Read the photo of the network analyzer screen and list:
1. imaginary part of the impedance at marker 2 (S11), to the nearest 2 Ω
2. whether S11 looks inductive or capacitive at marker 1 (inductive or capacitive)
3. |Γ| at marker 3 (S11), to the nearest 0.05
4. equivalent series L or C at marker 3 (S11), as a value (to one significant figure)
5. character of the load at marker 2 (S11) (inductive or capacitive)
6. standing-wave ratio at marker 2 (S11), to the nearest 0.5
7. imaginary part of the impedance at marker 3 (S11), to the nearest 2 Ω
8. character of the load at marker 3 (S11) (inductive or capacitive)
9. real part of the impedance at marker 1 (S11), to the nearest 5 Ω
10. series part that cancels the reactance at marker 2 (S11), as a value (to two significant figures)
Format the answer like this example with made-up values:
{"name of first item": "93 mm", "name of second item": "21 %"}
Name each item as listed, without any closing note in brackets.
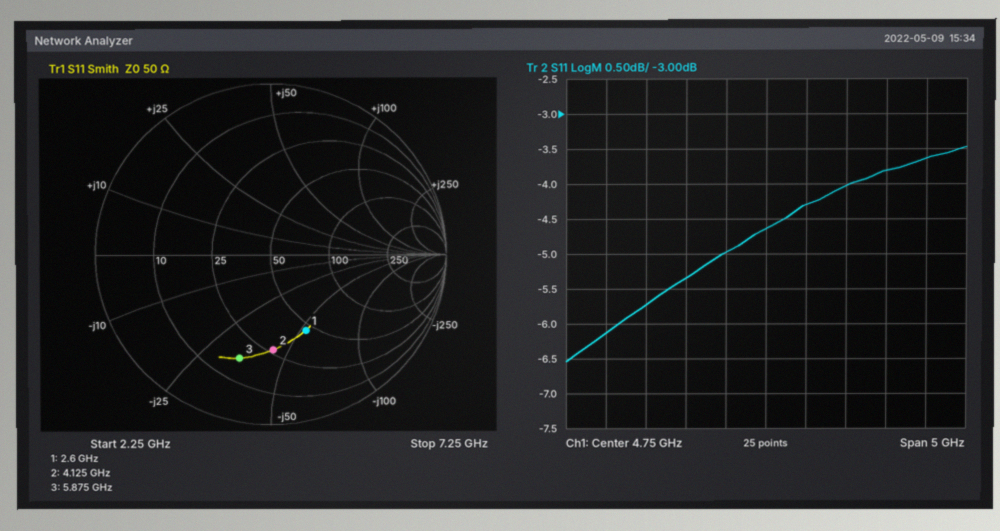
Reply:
{"imaginary part of the impedance at marker 2 (S11), to the nearest 2 Ω": "-44 Ω", "whether S11 looks inductive or capacitive at marker 1": "capacitive", "|Γ| at marker 3 (S11), to the nearest 0.05": "0.65", "equivalent series L or C at marker 3 (S11), as a value": "800 fF", "character of the load at marker 2 (S11)": "capacitive", "standing-wave ratio at marker 2 (S11), to the nearest 0.5": "3.5", "imaginary part of the impedance at marker 3 (S11), to the nearest 2 Ω": "-34 Ω", "character of the load at marker 3 (S11)": "capacitive", "real part of the impedance at marker 1 (S11), to the nearest 5 Ω": "45 Ω", "series part that cancels the reactance at marker 2 (S11), as a value": "1.7 nH"}
